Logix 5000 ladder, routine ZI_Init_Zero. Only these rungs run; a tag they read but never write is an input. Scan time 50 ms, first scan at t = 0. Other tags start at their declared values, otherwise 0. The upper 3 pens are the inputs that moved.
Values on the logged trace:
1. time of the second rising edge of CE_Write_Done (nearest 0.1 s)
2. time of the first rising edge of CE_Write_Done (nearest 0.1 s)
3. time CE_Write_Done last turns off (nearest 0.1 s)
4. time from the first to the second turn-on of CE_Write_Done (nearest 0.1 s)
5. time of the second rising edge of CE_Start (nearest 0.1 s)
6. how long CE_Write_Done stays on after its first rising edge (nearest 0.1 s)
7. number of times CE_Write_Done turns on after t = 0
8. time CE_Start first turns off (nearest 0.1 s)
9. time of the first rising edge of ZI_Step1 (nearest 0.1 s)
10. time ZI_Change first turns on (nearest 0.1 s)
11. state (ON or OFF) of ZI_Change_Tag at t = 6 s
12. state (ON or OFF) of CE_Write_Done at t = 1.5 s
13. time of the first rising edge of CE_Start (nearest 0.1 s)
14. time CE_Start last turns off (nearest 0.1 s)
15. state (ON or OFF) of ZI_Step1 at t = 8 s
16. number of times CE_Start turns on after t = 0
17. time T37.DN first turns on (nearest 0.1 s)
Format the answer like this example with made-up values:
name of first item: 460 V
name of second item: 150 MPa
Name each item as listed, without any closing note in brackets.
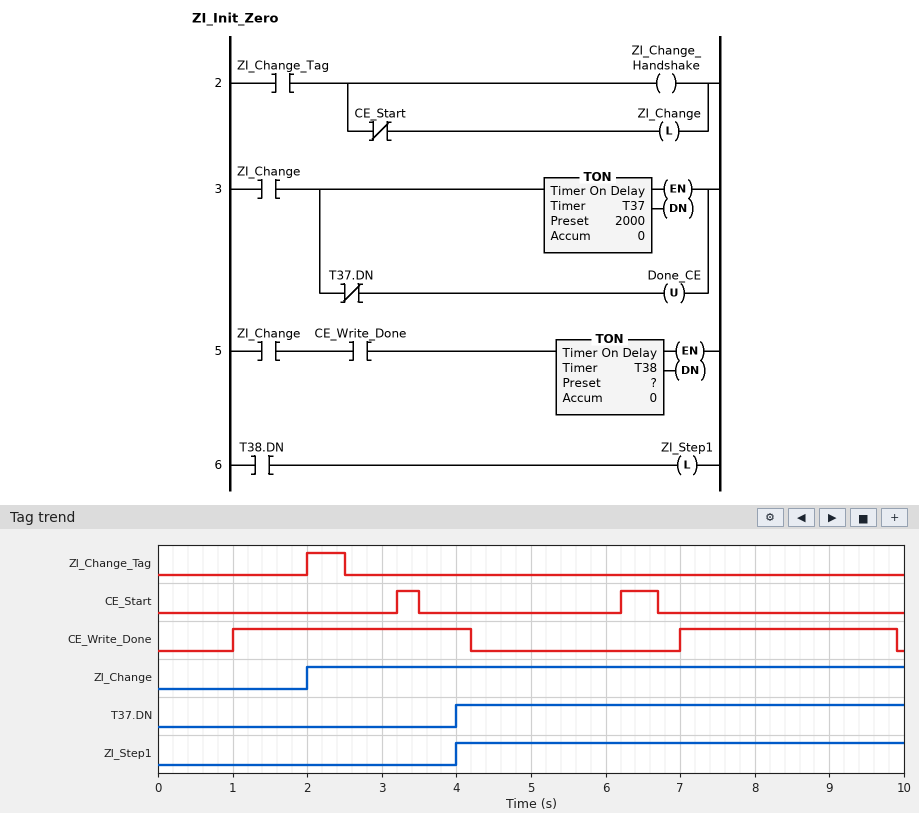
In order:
time of the second rising edge of CE_Write_Done: 7.0 s
time of the first rising edge of CE_Write_Done: 1.0 s
time CE_Write_Done last turns off: 9.9 s
time from the first to the second turn-on of CE_Write_Done: 6.0 s
time of the second rising edge of CE_Start: 6.2 s
how long CE_Write_Done stays on after its first rising edge: 3.2 s
number of times CE_Write_Done turns on after t = 0: 2
time CE_Start first turns off: 3.5 s
time of the first rising edge of ZI_Step1: 4.0 s
time ZI_Change first turns on: 2.0 s
state (ON or OFF) of ZI_Change_Tag at t = 6 s: OFF
state (ON or OFF) of CE_Write_Done at t = 1.5 s: ON
time of the first rising edge of CE_Start: 3.2 s
time CE_Start last turns off: 6.7 s
state (ON or OFF) of ZI_Step1 at t = 8 s: ON
number of times CE_Start turns on after t = 0: 2
time T37.DN first turns on: 4.0 s
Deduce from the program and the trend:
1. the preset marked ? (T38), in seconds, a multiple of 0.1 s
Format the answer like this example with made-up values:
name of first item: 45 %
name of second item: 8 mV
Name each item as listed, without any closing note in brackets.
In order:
the preset marked ? (T38), in seconds, a multiple of 0.1 s: 2.0 s
